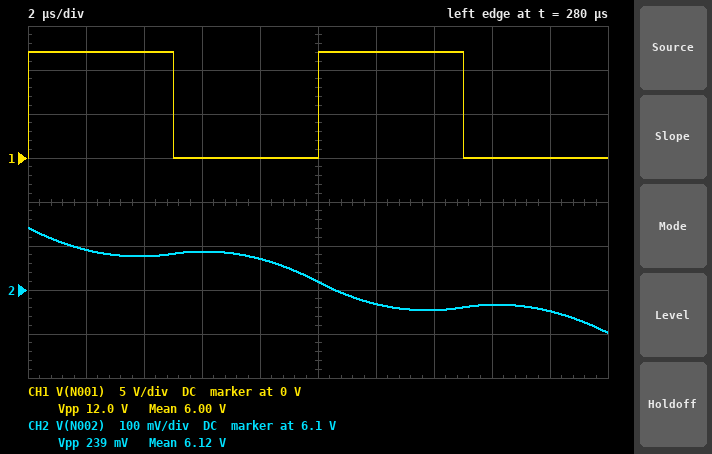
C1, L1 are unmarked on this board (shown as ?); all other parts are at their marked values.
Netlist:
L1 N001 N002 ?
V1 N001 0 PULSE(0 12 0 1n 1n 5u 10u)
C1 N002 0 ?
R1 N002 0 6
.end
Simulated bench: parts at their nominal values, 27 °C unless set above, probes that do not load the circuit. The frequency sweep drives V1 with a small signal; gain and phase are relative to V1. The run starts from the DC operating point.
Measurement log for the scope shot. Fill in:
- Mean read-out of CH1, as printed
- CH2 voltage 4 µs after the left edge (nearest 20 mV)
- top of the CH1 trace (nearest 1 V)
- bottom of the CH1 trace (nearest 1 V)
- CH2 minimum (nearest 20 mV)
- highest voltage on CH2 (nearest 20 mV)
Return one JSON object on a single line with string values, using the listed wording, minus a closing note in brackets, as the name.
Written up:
{"Mean read-out of CH1, as printed": "6.00 V", "CH2 voltage 4 µs after the left edge": "6.18 V", "top of the CH1 trace": "12 V", "bottom of the CH1 trace": "0 V", "CH2 minimum": "6.00 V", "highest voltage on CH2": "6.24 V"}
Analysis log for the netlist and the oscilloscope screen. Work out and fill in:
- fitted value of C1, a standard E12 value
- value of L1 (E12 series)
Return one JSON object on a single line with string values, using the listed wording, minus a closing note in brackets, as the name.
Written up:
{"fitted value of C1, a standard E12 value": "8.2 µF", "value of L1": "82 µH"}
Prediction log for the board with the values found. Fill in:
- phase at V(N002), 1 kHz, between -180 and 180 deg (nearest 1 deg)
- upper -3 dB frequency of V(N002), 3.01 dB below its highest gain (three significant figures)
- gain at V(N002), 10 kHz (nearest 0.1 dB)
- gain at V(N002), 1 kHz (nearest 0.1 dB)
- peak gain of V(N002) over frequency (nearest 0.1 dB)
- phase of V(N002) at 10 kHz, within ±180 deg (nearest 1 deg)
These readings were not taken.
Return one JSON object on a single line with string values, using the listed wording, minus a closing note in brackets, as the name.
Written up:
{"phase at V(N002), 1 kHz, between -180 and 180 deg": "-5 deg", "upper -3 dB frequency of V(N002), 3.01 dB below its highest gain": "7.18 kHz", "gain at V(N002), 10 kHz": "-5.4 dB", "gain at V(N002), 1 kHz": "0.2 dB", "peak gain of V(N002) over frequency": "5.9 dB", "phase of V(N002) at 10 kHz, within ±180 deg": "-153 deg"}
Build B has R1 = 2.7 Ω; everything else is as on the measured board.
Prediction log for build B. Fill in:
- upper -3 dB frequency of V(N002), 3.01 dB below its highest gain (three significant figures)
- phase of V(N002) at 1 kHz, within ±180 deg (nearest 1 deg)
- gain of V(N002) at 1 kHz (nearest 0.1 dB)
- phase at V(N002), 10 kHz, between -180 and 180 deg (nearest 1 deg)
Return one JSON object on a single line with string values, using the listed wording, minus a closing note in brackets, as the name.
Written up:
{"upper -3 dB frequency of V(N002), 3.01 dB below its highest gain": "6.90 kHz", "phase of V(N002) at 1 kHz, within ±180 deg": "-11 deg", "gain of V(N002) at 1 kHz": "0.1 dB", "phase at V(N002), 10 kHz, between -180 and 180 deg": "-131 deg"}
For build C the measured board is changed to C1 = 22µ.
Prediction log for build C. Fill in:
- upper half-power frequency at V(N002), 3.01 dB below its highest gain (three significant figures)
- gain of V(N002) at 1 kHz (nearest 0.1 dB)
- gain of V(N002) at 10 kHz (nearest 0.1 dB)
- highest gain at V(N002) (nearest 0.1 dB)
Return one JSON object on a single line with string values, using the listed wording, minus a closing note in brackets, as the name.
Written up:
{"upper half-power frequency at V(N002), 3.01 dB below its highest gain": "4.22 kHz", "gain of V(N002) at 1 kHz": "0.6 dB", "gain of V(N002) at 10 kHz": "-15.8 dB", "highest gain at V(N002)": "10.0 dB"}
